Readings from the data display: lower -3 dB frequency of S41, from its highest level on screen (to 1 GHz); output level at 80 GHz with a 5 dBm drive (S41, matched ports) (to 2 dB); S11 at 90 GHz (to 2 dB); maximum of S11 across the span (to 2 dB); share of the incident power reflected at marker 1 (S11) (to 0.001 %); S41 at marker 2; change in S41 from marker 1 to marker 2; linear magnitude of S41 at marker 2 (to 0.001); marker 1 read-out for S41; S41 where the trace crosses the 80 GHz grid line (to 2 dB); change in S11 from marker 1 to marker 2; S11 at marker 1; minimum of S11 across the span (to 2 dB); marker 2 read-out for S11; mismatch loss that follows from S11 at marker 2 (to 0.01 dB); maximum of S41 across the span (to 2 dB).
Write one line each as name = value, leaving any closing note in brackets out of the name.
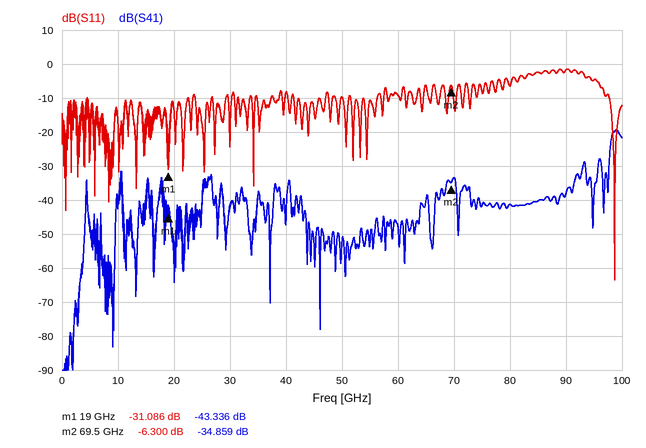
lower -3 dB frequency of S41, from its highest level on screen = 98 GHz
output level at 80 GHz with a 5 dBm drive (S41, matched ports) = -36 dBm
S11 at 90 GHz = -2 dB
maximum of S11 across the span = -2 dB
share of the incident power reflected at marker 1 (S11) = 0.078 %
S41 at marker 2 = -34.859 dB
change in S41 from marker 1 to marker 2 = 8.477 dB
linear magnitude of S41 at marker 2 = 0.018
marker 1 read-out for S41 = -43.336 dB
S41 where the trace crosses the 80 GHz grid line = -42 dB
change in S11 from marker 1 to marker 2 = 24.786 dB
S11 at marker 1 = -31.086 dB
minimum of S11 across the span = -64 dB
marker 2 read-out for S11 = -6.300 dB
mismatch loss that follows from S11 at marker 2 = 1.16 dB
maximum of S41 across the span = -20 dB
